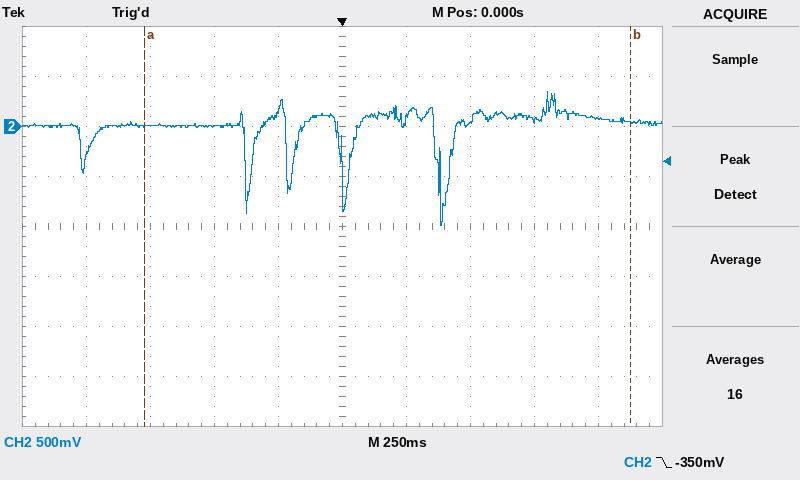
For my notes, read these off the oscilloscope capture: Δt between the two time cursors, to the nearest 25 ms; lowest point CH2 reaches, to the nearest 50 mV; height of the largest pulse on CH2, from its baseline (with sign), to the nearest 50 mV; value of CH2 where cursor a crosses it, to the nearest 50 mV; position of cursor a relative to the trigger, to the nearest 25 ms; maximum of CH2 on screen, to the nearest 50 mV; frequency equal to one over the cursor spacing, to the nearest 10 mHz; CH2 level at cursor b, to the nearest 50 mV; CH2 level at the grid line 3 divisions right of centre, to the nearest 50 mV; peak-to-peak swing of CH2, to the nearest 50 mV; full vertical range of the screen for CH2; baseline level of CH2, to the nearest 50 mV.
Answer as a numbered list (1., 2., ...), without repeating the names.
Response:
1. 1.900 s
2. -1.00 V
3. -1.00 V
4. 0 mV
5. -775 ms
6. 350 mV
7. 530 mHz
8. 50 mV
9. 50 mV
10. 1.35 V
11. 4 V
12. 0 mV
